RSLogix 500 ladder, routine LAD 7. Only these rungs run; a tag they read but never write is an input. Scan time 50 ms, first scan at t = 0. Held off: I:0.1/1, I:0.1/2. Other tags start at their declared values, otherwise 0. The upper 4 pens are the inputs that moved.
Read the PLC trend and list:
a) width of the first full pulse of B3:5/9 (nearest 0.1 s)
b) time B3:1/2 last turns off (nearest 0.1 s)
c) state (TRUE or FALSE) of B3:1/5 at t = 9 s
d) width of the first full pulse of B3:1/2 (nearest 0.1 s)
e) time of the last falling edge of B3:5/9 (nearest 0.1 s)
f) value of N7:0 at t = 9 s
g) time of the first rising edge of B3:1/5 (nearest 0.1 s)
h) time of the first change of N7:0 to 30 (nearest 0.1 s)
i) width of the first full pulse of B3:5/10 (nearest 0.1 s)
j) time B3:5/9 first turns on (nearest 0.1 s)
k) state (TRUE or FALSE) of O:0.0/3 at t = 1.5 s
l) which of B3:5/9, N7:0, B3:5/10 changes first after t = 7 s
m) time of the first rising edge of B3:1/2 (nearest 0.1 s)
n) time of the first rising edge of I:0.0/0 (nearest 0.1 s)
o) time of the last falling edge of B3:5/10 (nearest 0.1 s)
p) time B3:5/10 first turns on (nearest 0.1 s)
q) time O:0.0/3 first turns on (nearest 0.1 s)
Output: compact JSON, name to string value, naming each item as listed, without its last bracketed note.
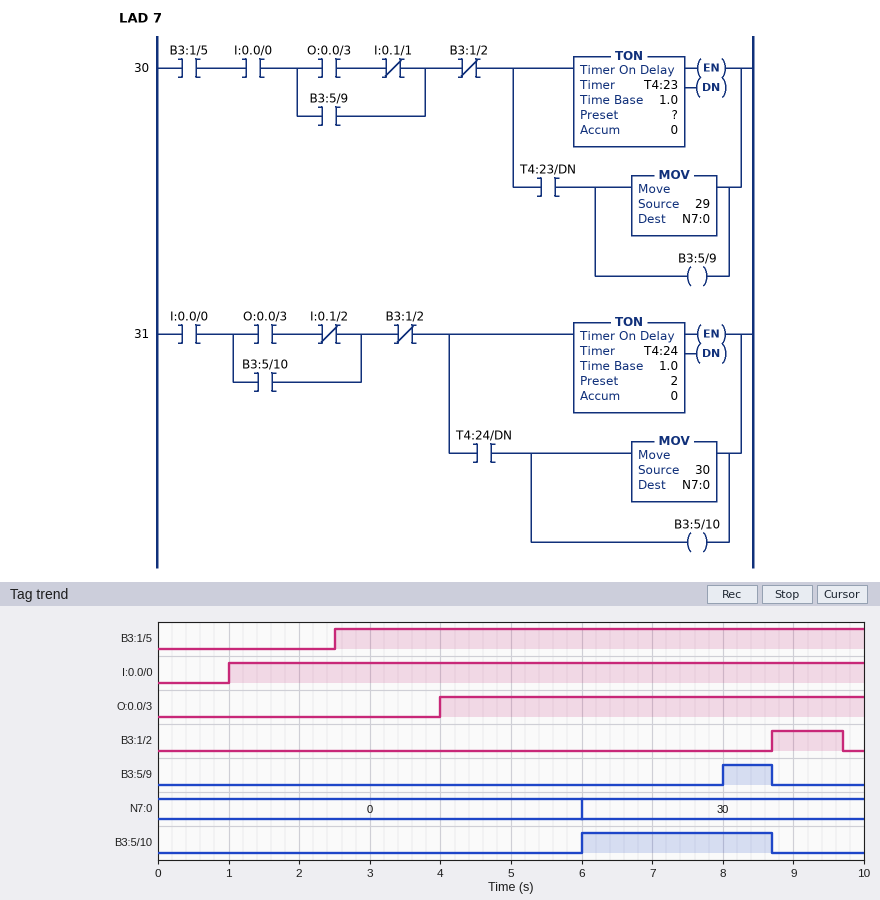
{"width of the first full pulse of B3:5/9": "0.7 s", "time B3:1/2 last turns off": "9.7 s", "state (TRUE or FALSE) of B3:1/5 at t = 9 s": "TRUE", "width of the first full pulse of B3:1/2": "1.0 s", "time of the last falling edge of B3:5/9": "8.7 s", "value of N7:0 at t = 9 s": "30", "time of the first rising edge of B3:1/5": "2.5 s", "time of the first change of N7:0 to 30": "6.0 s", "width of the first full pulse of B3:5/10": "2.7 s", "time B3:5/9 first turns on": "8.0 s", "state (TRUE or FALSE) of O:0.0/3 at t = 1.5 s": "FALSE", "which of B3:5/9, N7:0, B3:5/10 changes first after t = 7 s": "B3:5/9", "time of the first rising edge of B3:1/2": "8.7 s", "time of the first rising edge of I:0.0/0": "1.0 s", "time of the last falling edge of B3:5/10": "8.7 s", "time B3:5/10 first turns on": "6.0 s", "time O:0.0/3 first turns on": "4.0 s"}
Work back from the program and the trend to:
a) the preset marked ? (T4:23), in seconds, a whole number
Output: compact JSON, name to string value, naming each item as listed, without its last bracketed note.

{"the preset marked ? (T4:23), in seconds, a whole number": "4 s"}
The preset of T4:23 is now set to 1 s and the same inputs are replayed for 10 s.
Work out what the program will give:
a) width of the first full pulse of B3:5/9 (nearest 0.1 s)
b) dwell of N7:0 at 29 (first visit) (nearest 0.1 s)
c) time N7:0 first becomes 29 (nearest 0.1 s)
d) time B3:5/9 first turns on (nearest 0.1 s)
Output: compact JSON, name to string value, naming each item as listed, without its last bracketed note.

{"width of the first full pulse of B3:5/9": "3.7 s", "dwell of N7:0 at 29 (first visit)": "1.0 s", "time N7:0 first becomes 29": "5.0 s", "time B3:5/9 first turns on": "5.0 s"}
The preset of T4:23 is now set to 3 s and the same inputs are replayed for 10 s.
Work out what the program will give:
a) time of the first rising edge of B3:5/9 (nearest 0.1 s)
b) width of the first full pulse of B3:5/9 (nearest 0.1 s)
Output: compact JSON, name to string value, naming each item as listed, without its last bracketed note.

{"time of the first rising edge of B3:5/9": "7.0 s", "width of the first full pulse of B3:5/9": "1.7 s"}
